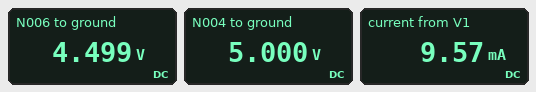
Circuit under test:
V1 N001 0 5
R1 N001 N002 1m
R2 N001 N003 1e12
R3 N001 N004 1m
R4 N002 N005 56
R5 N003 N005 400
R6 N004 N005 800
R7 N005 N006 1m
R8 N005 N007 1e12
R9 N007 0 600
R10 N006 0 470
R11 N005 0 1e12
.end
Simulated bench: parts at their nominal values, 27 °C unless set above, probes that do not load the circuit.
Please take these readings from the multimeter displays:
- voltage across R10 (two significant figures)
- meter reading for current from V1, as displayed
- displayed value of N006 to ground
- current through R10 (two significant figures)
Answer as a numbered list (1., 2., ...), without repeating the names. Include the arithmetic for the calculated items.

1. 4.499 V = 4.5 V
2. 9.57 mA
3. 4.499 V
4. (4.499 V) / 470 Ω = 9.6 mA
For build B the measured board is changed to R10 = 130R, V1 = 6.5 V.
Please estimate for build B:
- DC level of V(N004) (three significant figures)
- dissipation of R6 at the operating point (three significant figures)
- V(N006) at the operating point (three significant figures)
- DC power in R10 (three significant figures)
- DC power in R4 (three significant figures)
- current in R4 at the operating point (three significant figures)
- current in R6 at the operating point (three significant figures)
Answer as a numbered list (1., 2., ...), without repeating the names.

1. 6.50 V
2. 4.35 mW
3. 4.63 V
4. 165 mW
5. 62.2 mW
6. 33.3 mA
7. 2.33 mA
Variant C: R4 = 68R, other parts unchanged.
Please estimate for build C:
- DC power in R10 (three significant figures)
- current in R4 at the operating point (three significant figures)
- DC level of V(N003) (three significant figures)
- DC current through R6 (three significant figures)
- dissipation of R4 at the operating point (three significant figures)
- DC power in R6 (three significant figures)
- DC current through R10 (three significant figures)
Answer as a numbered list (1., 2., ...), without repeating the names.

1. 41.4 mW
2. 8.65 mA
3. 4.41 V
4. 735 µA
5. 5.09 mW
6. 433 µW
7. 9.39 mA
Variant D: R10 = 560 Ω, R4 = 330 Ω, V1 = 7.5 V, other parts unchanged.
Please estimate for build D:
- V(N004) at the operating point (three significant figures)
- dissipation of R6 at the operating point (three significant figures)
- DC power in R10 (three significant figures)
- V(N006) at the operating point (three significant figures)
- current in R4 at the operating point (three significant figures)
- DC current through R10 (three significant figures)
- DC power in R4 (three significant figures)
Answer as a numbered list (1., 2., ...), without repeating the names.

1. 7.50 V
2. 6.09 mW
3. 50.0 mW
4. 5.29 V
5. 6.69 mA
6. 9.45 mA
7. 14.8 mW
